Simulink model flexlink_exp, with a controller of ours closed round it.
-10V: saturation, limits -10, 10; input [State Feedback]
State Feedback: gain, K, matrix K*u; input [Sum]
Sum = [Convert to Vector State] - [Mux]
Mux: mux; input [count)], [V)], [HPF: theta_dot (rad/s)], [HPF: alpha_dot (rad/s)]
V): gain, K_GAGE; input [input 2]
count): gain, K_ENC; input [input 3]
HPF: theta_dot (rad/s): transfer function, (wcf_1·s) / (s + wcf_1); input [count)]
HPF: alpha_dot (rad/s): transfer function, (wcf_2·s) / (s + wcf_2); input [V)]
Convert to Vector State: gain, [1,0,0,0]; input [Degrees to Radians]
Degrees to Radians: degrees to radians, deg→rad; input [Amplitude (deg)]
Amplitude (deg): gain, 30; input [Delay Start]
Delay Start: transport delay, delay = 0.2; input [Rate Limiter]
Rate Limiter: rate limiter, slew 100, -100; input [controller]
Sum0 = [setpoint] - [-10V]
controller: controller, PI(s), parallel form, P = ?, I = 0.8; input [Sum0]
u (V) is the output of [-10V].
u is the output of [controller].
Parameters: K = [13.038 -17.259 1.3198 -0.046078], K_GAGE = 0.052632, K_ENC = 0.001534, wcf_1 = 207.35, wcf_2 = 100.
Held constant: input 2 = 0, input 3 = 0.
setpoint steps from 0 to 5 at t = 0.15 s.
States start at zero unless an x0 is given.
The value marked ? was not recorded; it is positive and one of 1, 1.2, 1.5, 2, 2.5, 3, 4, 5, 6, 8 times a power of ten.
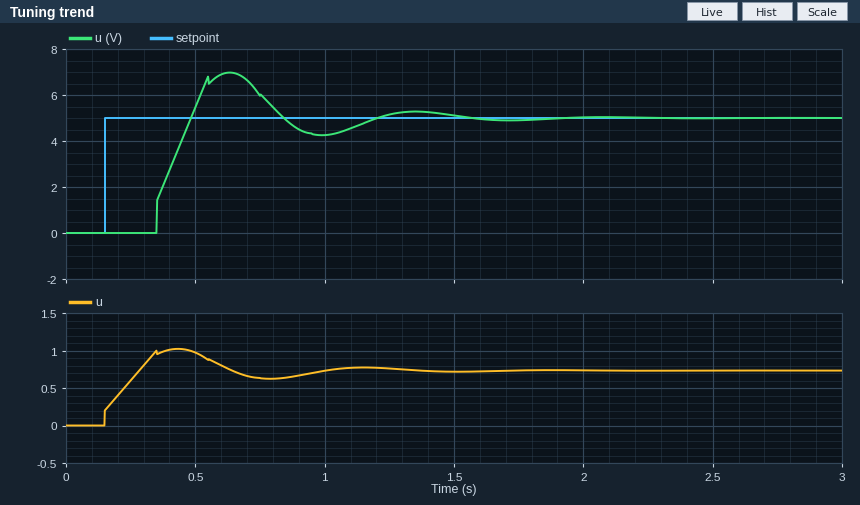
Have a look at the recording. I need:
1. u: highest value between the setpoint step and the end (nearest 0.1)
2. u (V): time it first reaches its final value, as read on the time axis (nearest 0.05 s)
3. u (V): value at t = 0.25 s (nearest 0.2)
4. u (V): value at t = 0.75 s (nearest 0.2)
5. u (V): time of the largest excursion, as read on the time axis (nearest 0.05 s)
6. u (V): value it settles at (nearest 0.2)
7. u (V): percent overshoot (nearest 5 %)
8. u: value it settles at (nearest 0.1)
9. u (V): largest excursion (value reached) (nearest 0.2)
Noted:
1.0
0.50 s
0.0
6.0
0.65 s
5.0
40 %
0.7
7.0
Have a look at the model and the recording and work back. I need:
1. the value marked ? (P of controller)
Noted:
0.04
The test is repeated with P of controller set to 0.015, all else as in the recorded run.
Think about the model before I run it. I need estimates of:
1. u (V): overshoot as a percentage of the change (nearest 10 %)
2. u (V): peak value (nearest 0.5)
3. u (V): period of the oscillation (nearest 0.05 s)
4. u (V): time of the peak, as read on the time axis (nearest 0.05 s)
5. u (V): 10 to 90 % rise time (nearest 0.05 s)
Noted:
50 %
7.5
0.85 s
0.70 s
0.15 s
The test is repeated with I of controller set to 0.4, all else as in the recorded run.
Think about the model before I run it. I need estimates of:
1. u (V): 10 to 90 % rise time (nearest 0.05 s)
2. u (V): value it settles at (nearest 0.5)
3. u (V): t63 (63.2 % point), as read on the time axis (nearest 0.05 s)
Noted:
0.50 s
5.0
0.50 s
